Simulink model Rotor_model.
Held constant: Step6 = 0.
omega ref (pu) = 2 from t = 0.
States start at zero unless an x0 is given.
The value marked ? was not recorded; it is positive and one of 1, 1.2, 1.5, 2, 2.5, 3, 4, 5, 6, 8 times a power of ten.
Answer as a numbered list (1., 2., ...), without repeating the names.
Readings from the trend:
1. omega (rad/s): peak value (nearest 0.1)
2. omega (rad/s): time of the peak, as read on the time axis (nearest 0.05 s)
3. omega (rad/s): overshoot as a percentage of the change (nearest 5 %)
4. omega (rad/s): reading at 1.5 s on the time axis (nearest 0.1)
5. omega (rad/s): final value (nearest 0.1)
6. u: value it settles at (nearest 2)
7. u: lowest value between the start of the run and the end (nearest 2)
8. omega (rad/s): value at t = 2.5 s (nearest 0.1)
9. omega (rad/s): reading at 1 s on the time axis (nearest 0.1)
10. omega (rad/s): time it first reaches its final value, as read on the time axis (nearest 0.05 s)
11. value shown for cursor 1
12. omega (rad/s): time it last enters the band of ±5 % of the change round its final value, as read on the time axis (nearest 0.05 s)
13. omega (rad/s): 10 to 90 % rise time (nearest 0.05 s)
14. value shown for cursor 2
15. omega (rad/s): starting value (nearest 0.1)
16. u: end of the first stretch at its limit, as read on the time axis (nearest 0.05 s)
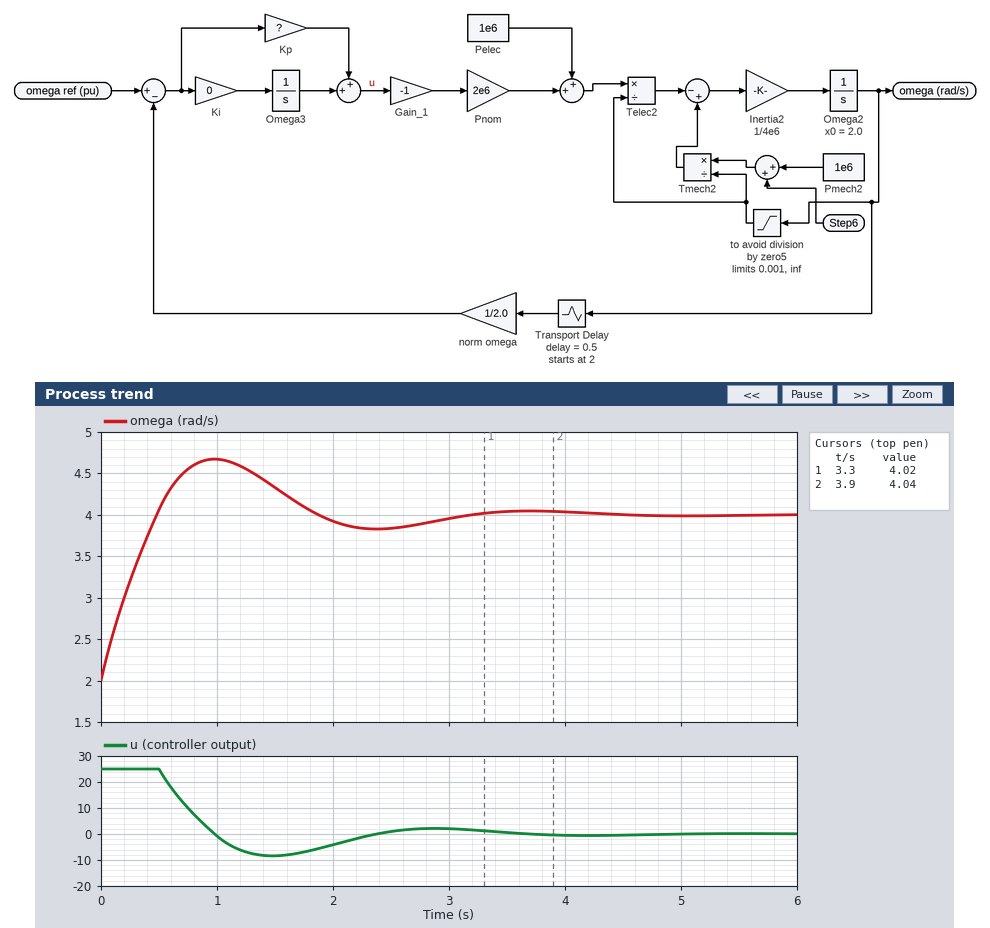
1. 4.7
2. 1.00 s
3. 35 %
4. 4.3
5. 4.0
6. 0
7. -8
8. 3.8
9. 4.7
10. 0.50 s
11. 4.02
12. 2.80 s
13. 0.40 s
14. 4.04
15. 2.0
16. 0.50 s
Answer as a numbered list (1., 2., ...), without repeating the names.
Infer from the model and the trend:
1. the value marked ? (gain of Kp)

1. 25
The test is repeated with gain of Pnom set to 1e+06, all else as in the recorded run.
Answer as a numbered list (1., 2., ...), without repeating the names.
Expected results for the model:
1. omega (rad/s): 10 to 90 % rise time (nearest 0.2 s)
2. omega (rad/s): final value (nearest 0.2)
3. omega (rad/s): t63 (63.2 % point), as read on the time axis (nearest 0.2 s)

1. 1.0 s
2. 4.0
3. 0.6 s
